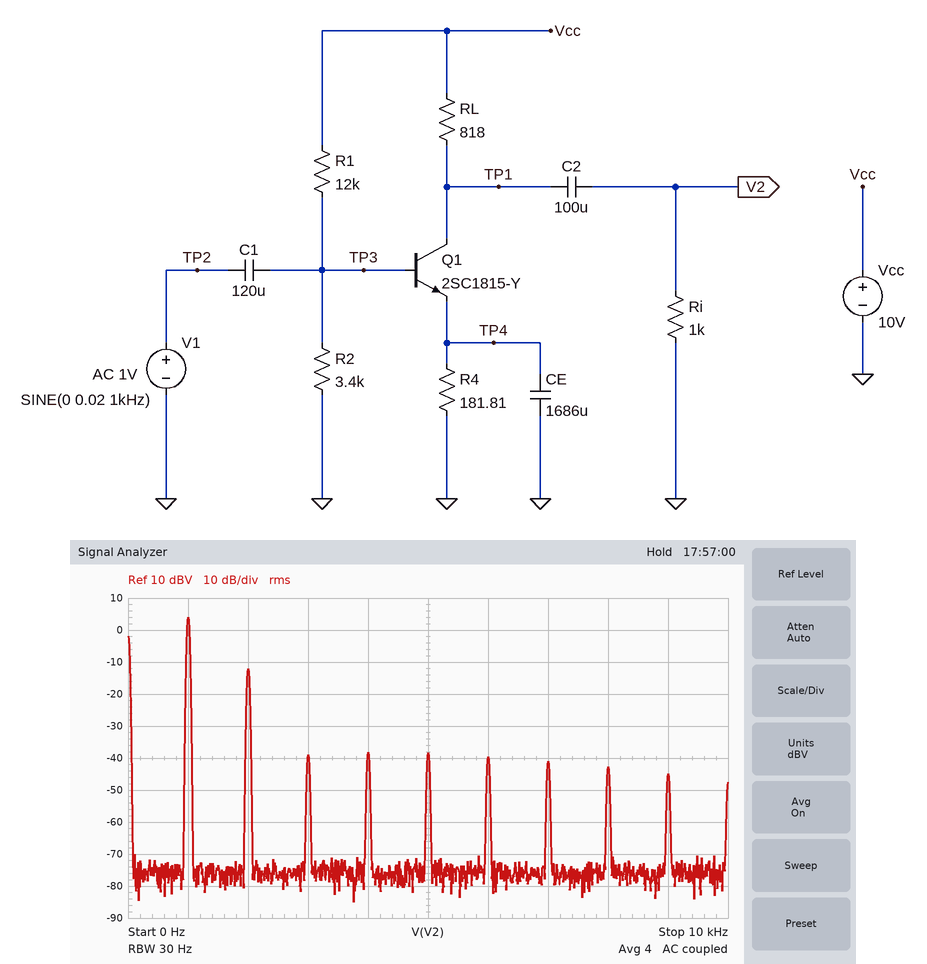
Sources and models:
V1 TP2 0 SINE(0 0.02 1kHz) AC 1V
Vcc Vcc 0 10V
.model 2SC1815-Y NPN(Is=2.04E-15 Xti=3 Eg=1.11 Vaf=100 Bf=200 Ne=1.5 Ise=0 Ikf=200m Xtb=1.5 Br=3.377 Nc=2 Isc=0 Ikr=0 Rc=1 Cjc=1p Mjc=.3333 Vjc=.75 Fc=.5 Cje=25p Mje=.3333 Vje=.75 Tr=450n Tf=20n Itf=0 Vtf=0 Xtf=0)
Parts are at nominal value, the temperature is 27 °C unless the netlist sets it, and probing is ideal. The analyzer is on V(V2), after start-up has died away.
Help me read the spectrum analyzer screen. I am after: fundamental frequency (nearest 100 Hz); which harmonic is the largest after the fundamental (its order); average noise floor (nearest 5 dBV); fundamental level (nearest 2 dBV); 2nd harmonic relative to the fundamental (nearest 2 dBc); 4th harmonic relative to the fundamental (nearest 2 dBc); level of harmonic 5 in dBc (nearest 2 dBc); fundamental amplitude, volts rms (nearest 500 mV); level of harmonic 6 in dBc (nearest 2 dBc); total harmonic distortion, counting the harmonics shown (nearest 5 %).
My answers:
1.0 kHz
2
-75 dBV
4 dBV
-16 dBc
-42 dBc
-42 dBc
1.5 V
-44 dBc
15 %
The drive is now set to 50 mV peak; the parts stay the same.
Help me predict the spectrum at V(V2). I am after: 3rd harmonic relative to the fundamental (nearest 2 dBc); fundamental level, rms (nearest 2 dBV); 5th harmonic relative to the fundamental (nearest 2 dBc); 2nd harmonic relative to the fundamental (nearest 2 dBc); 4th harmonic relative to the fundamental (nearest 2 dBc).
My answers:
-38 dBc
8 dBV
-26 dBc
-10 dBc
-24 dBc
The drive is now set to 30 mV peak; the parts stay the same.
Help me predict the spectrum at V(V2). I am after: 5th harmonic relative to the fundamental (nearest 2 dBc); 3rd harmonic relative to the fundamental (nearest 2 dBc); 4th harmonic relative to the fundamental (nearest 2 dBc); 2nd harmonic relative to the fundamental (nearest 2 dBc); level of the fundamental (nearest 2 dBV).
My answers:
-30 dBc
-38 dBc
-28 dBc
-14 dBc
6 dBV
